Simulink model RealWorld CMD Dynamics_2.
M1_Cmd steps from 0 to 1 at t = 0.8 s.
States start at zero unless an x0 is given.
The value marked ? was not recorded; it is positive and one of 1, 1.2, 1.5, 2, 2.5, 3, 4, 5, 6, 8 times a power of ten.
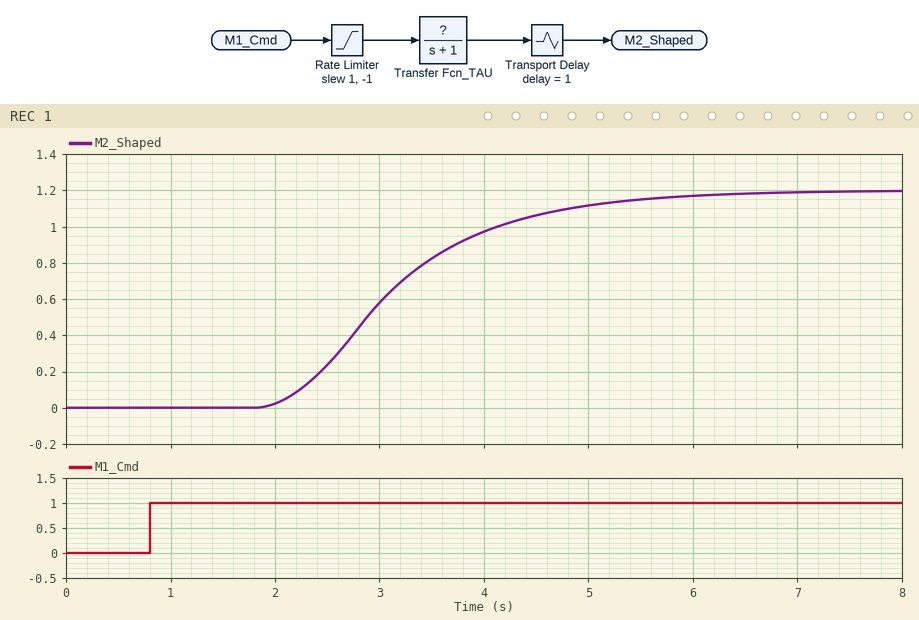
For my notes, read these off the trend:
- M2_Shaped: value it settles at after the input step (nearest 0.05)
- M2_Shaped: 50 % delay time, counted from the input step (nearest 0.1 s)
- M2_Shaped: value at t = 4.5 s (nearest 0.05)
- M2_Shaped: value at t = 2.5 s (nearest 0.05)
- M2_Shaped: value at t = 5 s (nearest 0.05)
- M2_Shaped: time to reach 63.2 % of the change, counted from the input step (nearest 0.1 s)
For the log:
1.20
2.2 s
1.05
0.25
1.10
2.5 s
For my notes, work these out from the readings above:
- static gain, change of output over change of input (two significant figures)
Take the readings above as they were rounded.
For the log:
1.2
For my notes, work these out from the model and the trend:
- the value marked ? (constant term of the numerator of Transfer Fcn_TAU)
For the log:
1.2
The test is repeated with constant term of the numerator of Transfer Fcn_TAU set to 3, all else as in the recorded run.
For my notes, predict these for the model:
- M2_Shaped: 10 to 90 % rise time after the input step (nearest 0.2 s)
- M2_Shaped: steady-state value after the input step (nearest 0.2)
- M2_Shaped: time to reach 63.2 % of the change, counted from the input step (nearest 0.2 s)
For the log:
2.4 s
3.0
2.6 s
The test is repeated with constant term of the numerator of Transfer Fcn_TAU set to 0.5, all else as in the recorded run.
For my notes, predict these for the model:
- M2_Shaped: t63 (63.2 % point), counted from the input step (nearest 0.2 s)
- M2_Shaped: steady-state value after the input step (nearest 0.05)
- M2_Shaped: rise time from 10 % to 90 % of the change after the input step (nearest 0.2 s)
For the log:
2.6 s
0.50
2.4 s
